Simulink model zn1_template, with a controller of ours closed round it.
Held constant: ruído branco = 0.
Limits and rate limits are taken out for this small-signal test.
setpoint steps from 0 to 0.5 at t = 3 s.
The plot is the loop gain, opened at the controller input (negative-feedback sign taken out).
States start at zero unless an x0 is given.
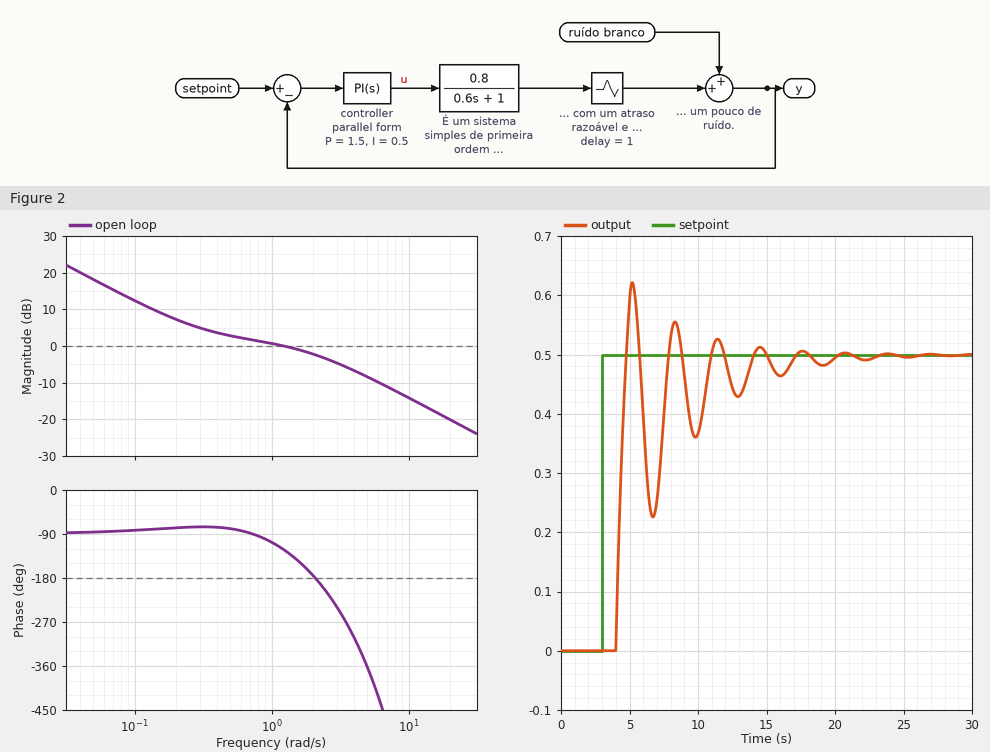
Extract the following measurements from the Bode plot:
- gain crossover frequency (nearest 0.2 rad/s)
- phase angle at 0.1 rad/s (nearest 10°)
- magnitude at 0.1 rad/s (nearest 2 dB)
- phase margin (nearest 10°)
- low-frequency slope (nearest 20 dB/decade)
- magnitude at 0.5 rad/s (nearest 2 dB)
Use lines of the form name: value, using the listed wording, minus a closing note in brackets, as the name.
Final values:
gain crossover frequency: 1.2 rad/s
phase angle at 0.1 rad/s: -80°
magnitude at 0.1 rad/s: 12 dB
phase margin: 60°
low-frequency slope: -20 dB/decade
magnitude at 0.5 rad/s: 2 dB
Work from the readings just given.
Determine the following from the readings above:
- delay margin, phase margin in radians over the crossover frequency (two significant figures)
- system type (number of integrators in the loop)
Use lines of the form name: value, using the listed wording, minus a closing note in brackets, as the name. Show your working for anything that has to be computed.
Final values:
delay margin, phase margin in radians over the crossover frequency: 60 × π / 180 / 1.2 = 0.87 s
system type: 1
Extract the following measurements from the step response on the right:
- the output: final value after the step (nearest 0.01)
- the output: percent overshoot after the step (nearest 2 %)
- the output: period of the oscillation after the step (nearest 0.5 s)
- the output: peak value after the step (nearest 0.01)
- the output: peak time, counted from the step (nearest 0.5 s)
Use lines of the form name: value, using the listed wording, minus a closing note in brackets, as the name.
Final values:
the output: final value after the step: 0.50
the output: percent overshoot after the step: 24 %
the output: period of the oscillation after the step: 3.0 s
the output: peak value after the step: 0.62
the output: peak time, counted from the step: 2.0 s
